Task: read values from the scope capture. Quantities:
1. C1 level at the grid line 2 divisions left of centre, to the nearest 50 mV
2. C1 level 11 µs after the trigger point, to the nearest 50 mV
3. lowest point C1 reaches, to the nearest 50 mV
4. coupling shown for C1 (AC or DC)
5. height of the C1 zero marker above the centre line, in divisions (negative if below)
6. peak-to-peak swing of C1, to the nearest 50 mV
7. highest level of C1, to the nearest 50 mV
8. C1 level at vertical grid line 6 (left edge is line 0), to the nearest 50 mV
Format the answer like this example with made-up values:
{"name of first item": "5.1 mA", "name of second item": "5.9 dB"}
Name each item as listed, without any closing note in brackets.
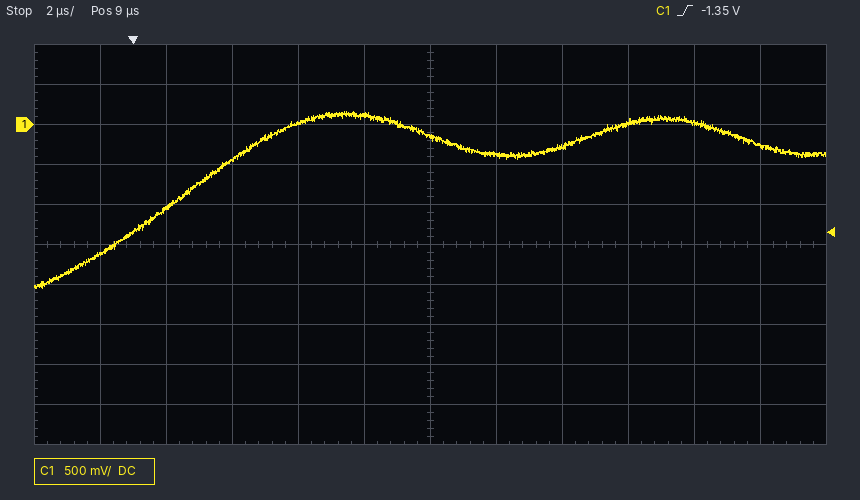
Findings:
{"C1 level at the grid line 2 divisions left of centre, to the nearest 50 mV": "0 mV", "C1 level 11 µs after the trigger point, to the nearest 50 mV": "-350 mV", "lowest point C1 reaches, to the nearest 50 mV": "-2.05 V", "coupling shown for C1": "DC", "height of the C1 zero marker above the centre line, in divisions": "+3.0 div", "peak-to-peak swing of C1, to the nearest 50 mV": "2.20 V", "highest level of C1, to the nearest 50 mV": "150 mV", "C1 level at vertical grid line 6 (left edge is line 0), to the nearest 50 mV": "-150 mV"}
